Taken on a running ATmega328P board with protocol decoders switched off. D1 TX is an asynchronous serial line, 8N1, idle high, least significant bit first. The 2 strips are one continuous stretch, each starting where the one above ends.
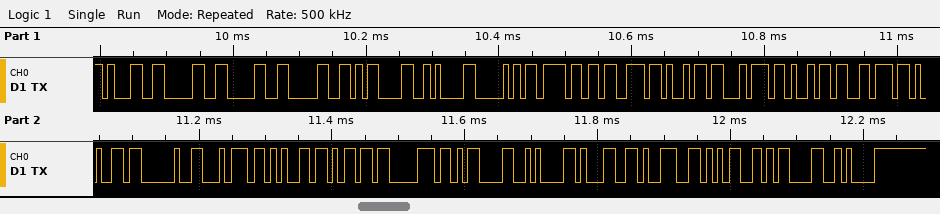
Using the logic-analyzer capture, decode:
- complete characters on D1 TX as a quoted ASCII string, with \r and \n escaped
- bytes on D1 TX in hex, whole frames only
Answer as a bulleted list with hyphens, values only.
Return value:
- "1000\r\nPositive temp\r\n195\r\n"
- 31 30 30 30 0D 0A 50 6F 73 69 74 69 76 65 20 74 65 6D 70 0D 0A 31 39 35 0D 0A
